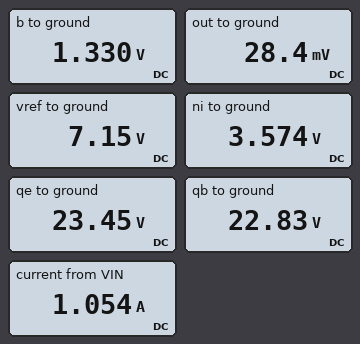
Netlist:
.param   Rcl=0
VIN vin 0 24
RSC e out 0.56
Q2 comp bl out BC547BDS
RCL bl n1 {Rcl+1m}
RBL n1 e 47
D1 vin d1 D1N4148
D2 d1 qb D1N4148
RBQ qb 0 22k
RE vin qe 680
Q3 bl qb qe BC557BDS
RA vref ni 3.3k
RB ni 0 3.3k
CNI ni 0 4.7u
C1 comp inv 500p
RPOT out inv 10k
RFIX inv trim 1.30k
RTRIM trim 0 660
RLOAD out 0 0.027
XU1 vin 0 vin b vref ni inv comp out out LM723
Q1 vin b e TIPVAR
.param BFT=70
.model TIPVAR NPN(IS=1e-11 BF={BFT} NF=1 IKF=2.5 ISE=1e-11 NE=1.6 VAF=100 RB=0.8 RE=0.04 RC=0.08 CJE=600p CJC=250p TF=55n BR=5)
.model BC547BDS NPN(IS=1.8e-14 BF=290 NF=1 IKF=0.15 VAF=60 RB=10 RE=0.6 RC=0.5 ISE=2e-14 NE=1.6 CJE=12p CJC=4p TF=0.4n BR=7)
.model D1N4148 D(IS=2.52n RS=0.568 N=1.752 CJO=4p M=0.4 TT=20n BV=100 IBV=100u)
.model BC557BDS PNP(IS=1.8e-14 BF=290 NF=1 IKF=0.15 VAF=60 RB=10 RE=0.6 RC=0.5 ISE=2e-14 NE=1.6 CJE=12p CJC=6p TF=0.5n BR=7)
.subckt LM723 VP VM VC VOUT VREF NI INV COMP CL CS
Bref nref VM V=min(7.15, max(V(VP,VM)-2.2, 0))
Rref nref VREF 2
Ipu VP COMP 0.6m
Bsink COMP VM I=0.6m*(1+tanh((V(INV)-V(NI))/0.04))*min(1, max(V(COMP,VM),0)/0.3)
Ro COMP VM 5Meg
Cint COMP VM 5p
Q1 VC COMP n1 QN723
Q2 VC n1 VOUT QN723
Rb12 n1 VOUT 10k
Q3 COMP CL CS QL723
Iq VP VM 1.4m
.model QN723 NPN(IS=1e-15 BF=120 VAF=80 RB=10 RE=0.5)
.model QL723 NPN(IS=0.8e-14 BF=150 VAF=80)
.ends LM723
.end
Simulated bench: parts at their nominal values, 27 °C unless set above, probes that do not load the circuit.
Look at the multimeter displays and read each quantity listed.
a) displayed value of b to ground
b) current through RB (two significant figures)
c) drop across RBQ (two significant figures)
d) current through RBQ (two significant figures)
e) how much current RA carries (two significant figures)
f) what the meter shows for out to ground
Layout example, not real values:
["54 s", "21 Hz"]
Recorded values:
["1.330 V", "1.1 mA", "23 V", "1.0 mA", "1.1 mA", "28.4 mV"]
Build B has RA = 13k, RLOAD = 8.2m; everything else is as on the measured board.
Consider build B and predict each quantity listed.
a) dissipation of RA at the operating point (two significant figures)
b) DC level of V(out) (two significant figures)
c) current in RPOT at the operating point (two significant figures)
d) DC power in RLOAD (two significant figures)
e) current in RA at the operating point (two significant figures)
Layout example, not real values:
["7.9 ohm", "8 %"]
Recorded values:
["2.5 mW", "8.6 mV", "720 nA", "9.1 mW", "440 µA"]
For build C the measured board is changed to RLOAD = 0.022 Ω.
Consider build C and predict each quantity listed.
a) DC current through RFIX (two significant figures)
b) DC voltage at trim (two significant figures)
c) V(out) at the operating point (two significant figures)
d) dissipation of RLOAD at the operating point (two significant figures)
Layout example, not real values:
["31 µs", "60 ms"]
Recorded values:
["1.9 µA", "1.3 mV", "23 mV", "24 mW"]
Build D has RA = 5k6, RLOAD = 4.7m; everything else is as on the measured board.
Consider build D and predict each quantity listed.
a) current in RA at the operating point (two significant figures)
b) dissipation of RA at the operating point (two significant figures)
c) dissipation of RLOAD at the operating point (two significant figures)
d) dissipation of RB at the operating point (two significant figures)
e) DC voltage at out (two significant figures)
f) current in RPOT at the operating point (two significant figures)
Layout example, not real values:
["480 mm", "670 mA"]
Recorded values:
["800 µA", "3.6 mW", "5.2 mW", "2.1 mW", "4.9 mV", "410 nA"]
